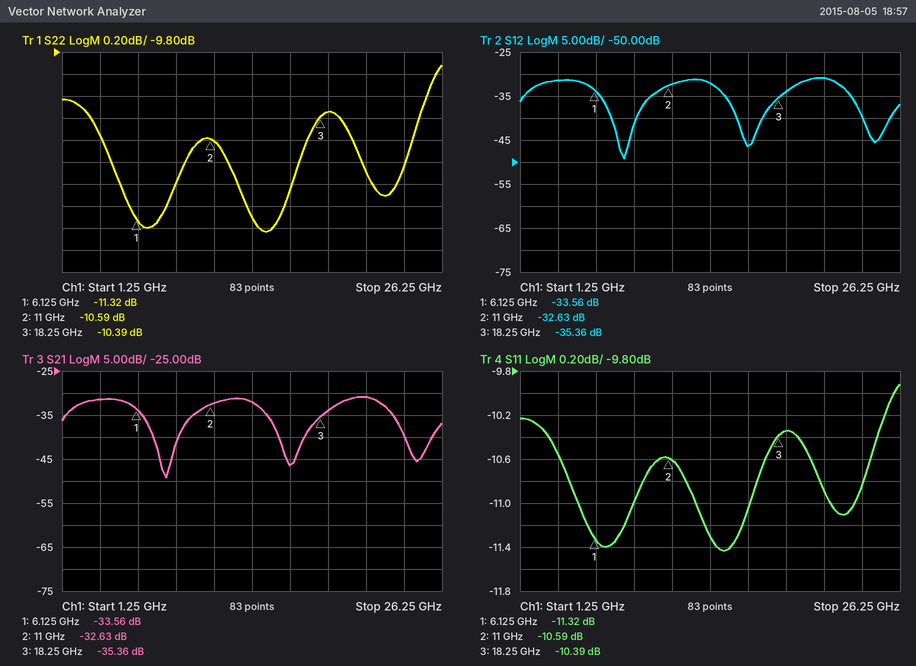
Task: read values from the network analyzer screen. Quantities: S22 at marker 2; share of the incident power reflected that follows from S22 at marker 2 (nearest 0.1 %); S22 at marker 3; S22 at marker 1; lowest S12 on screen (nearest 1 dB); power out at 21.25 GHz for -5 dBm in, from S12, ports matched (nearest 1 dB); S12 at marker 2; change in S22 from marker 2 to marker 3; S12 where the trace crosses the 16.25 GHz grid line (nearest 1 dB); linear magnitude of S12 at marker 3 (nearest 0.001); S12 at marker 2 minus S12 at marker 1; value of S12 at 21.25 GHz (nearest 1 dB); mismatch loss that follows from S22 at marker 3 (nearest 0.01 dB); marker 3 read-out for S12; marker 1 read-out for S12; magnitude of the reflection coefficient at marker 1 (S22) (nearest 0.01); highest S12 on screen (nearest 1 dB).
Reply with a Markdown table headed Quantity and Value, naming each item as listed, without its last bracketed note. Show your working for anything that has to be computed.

| Quantity | Value |
|---|---|
| S22 at marker 2 | -10.59 dB |
| share of the incident power reflected that follows from S22 at marker 2 | 10^(-10.59/10) ≈ 8.7 % |
| S22 at marker 3 | -10.39 dB |
| S22 at marker 1 | -11.32 dB |
| lowest S12 on screen | -49 dB |
| power out at 21.25 GHz for -5 dBm in, from S12, ports matched | -5 dBm + (-31 dB) = -36 dBm |
| S12 at marker 2 | -32.63 dB |
| change in S22 from marker 2 to marker 3 | -10.39 − (-10.59) = 0.20 dB |
| S12 where the trace crosses the 16.25 GHz grid line | -46 dB |
| linear magnitude of S12 at marker 3 | 10^(-35.36/20) ≈ 0.017 |
| S12 at marker 2 minus S12 at marker 1 | -32.63 − (-33.56) = 0.93 dB |
| value of S12 at 21.25 GHz | -31 dB |
| mismatch loss that follows from S22 at marker 3 | −10 log10(1 − 10^(-10.39/10)) ≈ 0.42 dB |
| marker 3 read-out for S12 | -35.36 dB |
| marker 1 read-out for S12 | -33.56 dB |
| magnitude of the reflection coefficient at marker 1 (S22) | 10^(-11.32/20) ≈ 0.27 |
| highest S12 on screen | -31 dB |
